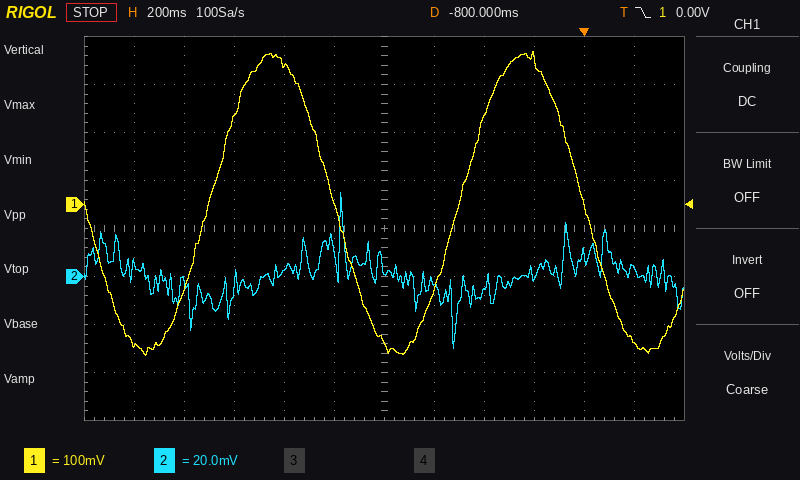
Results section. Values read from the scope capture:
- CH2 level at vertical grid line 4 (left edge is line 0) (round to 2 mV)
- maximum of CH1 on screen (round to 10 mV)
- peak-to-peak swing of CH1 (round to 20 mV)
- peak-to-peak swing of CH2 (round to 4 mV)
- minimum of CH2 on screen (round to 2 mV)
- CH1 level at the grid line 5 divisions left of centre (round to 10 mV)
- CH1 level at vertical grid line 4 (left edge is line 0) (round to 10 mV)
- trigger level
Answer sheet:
2 mV
320 mV
640 mV
64 mV
-30 mV
-290 mV
290 mV
0.00 V
